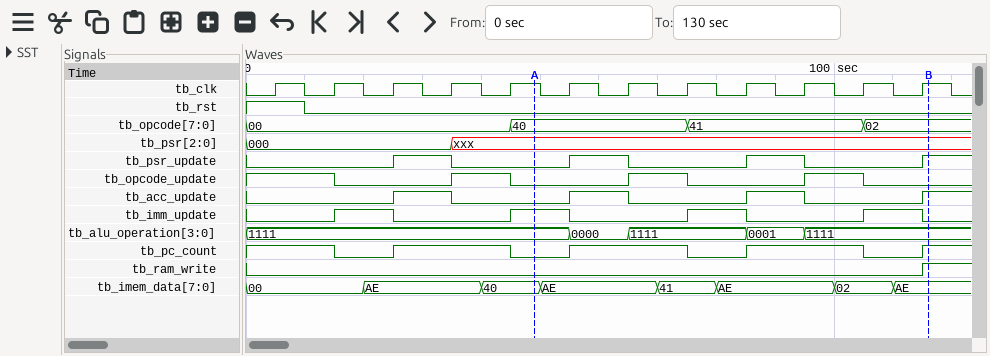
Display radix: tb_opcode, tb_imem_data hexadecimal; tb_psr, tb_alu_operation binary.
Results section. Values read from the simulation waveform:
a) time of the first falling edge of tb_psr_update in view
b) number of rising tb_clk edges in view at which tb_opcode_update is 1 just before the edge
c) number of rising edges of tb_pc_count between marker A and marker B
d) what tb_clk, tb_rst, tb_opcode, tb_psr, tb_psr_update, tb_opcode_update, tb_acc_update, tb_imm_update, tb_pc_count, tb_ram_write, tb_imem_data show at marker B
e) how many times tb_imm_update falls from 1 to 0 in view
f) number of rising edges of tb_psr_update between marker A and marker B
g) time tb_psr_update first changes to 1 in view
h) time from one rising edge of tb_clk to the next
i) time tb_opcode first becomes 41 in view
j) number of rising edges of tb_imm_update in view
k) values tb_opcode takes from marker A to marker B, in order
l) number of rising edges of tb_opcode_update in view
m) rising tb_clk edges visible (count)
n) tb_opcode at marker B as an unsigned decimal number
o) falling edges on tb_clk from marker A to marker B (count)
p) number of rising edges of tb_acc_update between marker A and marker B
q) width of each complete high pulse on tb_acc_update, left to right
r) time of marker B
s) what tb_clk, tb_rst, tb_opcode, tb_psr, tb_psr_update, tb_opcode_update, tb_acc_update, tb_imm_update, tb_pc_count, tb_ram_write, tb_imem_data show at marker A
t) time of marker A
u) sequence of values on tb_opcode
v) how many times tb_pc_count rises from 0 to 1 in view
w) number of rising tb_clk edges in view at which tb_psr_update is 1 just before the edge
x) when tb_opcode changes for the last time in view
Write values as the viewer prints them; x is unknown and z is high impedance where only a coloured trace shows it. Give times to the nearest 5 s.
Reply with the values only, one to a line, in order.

35 s
5
3
tb_clk=1, tb_rst=0, tb_opcode=02, tb_psr=xxx, tb_psr_update=1, tb_opcode_update=0, tb_acc_update=1, tb_imm_update=0, tb_pc_count=1, tb_ram_write=1, tb_imem_data=AE
4
3
25 s
10 s
75 s
4
40, 41, 02
3
12
2
7
3
10 s, 10 s, 10 s
115 s
tb_clk=1, tb_rst=0, tb_opcode=40, tb_psr=xxx, tb_psr_update=0, tb_opcode_update=0, tb_acc_update=0, tb_imm_update=1, tb_pc_count=0, tb_ram_write=0, tb_imem_data=40
50 s
00, 40, 41, 02
4
3
105 s
